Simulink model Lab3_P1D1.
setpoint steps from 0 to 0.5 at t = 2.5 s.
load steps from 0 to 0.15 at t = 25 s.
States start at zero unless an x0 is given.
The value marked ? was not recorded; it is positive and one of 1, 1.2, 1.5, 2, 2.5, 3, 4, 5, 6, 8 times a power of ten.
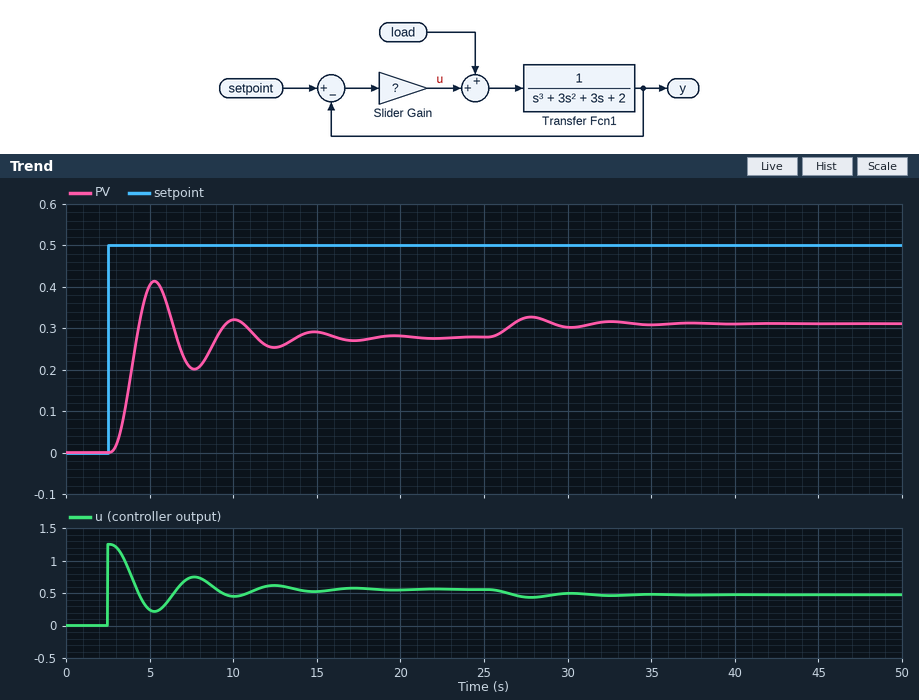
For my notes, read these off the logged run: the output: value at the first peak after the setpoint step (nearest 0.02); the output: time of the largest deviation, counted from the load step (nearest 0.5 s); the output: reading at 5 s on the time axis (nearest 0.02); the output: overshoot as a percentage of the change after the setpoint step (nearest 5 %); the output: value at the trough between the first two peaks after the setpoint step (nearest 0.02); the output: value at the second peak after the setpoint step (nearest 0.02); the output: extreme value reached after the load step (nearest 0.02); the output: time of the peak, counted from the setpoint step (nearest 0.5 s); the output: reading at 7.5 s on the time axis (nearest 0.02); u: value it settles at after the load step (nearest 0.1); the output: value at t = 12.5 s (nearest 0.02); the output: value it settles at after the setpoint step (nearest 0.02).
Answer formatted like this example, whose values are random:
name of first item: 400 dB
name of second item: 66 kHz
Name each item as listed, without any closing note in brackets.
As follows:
the output: value at the first peak after the setpoint step: 0.42
the output: time of the largest deviation, counted from the load step: 3.0 s
the output: reading at 5 s on the time axis: 0.40
the output: overshoot as a percentage of the change after the setpoint step: 50 %
the output: value at the trough between the first two peaks after the setpoint step: 0.20
the output: value at the second peak after the setpoint step: 0.32
the output: extreme value reached after the load step: 0.32
the output: time of the peak, counted from the setpoint step: 3.0 s
the output: reading at 7.5 s on the time axis: 0.20
u: value it settles at after the load step: 0.5
the output: value at t = 12.5 s: 0.26
the output: value it settles at after the setpoint step: 0.28
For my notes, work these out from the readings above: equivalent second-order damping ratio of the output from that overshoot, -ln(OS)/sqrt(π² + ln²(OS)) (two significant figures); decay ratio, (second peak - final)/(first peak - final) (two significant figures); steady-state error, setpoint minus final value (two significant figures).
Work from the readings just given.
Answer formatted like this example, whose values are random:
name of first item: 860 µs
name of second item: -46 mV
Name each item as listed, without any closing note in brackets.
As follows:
equivalent second-order damping ratio of the output from that overshoot, -ln(OS)/sqrt(π² + ln²(OS)): 0.22
decay ratio, (second peak - final)/(first peak - final): 0.29
steady-state error, setpoint minus final value: 0.22
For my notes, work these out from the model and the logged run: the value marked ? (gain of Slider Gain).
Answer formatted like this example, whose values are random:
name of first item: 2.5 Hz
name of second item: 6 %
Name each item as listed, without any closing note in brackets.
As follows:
the value marked ?: 2.5
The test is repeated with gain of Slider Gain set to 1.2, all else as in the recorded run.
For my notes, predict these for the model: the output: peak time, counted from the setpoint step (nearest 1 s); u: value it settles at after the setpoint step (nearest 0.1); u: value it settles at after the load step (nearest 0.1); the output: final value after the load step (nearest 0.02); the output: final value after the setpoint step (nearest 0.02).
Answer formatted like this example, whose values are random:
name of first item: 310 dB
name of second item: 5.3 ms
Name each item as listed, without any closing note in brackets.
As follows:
the output: peak time, counted from the setpoint step: 3 s
u: value it settles at after the setpoint step: 0.4
u: value it settles at after the load step: 0.3
the output: final value after the load step: 0.24
the output: final value after the setpoint step: 0.18
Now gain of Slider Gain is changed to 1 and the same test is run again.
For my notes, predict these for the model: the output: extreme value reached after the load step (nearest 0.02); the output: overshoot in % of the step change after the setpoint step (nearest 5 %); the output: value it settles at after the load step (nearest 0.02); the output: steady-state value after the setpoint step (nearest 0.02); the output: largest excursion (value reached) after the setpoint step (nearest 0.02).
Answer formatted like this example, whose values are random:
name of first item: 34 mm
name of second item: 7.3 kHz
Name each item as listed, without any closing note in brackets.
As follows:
the output: extreme value reached after the load step: 0.24
the output: overshoot in % of the step change after the setpoint step: 30 %
the output: value it settles at after the load step: 0.22
the output: steady-state value after the setpoint step: 0.16
the output: largest excursion (value reached) after the setpoint step: 0.22
